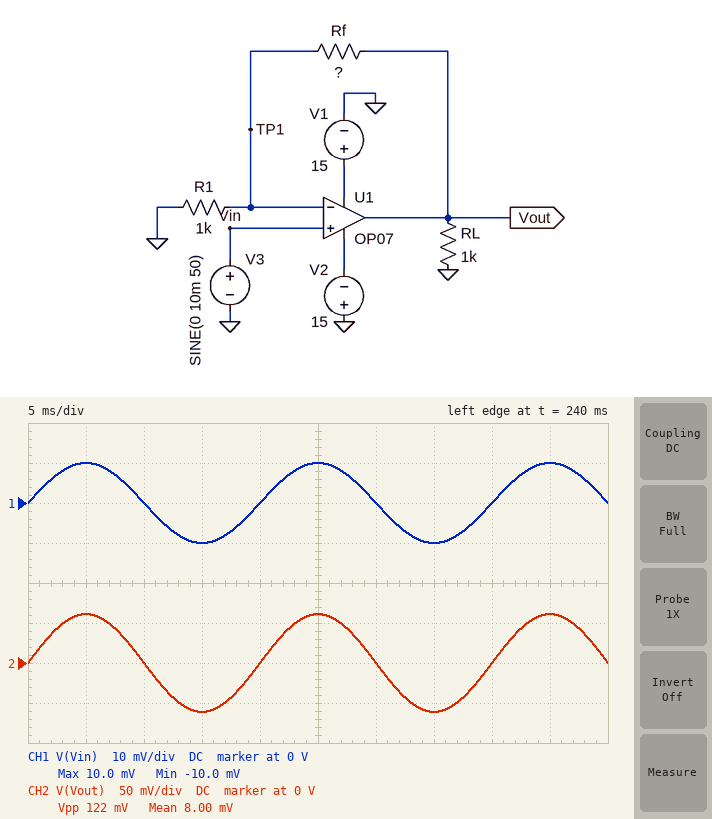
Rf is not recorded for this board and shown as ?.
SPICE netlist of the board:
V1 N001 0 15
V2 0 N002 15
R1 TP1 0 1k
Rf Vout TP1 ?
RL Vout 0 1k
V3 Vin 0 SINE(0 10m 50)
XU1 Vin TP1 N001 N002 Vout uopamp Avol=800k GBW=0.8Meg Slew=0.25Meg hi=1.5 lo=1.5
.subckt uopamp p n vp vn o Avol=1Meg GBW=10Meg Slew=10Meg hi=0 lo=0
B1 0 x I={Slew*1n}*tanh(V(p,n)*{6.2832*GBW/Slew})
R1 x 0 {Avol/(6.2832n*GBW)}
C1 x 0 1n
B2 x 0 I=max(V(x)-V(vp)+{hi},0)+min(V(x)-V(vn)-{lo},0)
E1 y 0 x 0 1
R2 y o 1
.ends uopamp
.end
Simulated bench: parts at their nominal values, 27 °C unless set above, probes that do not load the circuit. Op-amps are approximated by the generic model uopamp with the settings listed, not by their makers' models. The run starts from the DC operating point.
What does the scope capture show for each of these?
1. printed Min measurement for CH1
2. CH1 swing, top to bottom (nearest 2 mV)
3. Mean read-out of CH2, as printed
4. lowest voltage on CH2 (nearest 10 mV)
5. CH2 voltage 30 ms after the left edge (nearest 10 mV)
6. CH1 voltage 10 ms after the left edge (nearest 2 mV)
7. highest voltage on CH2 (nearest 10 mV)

-10.0 mV
20 mV
8.00 mV
-60 mV
0 V
0 V
60 mV
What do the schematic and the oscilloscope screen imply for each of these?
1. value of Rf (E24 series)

5.1 kΩ
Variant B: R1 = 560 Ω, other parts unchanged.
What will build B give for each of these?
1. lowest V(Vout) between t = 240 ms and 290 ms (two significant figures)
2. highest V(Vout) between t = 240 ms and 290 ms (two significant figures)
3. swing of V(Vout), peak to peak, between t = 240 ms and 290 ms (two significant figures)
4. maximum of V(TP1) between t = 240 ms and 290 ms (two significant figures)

-100 mV
100 mV
200 mV
10 mV
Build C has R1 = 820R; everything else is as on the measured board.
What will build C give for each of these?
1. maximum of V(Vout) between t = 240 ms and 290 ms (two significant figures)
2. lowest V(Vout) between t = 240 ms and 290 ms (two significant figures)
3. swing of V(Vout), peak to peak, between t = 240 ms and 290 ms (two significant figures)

72 mV
-72 mV
140 mV
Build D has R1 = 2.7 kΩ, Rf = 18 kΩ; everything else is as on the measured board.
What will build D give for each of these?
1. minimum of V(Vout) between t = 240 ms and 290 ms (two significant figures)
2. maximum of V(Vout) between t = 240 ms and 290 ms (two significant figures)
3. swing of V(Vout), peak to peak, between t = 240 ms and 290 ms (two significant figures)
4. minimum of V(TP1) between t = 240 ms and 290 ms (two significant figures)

-77 mV
77 mV
150 mV
-10 mV
